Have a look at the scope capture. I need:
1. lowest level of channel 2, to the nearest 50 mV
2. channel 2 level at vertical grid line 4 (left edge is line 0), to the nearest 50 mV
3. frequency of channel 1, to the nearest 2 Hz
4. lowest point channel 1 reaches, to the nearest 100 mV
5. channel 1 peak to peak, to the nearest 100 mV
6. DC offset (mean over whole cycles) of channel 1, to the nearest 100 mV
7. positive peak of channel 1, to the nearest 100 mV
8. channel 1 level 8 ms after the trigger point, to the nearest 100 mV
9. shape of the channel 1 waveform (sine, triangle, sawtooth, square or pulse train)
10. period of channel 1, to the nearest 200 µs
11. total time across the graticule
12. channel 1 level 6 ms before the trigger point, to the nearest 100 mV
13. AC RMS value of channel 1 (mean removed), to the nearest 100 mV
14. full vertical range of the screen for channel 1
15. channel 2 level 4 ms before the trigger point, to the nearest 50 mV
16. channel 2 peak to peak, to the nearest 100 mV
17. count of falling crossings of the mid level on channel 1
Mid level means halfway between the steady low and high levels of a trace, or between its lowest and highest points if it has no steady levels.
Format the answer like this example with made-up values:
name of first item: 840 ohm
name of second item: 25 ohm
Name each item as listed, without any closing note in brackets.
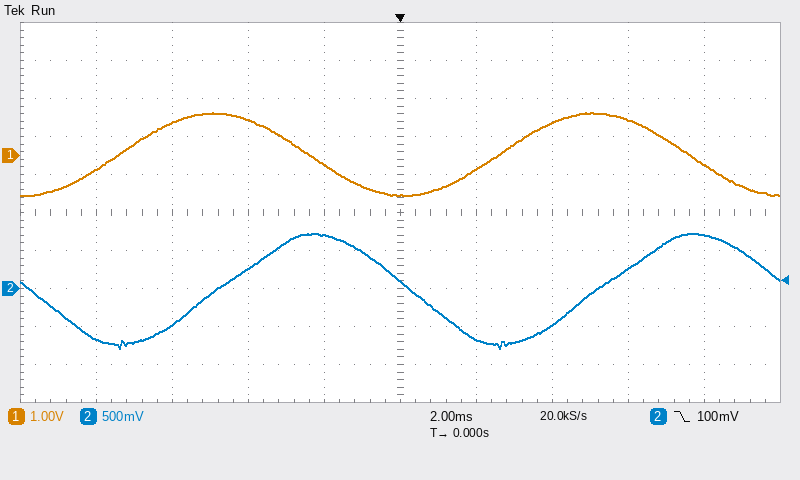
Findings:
lowest level of channel 2, to the nearest 50 mV: -800 mV
channel 2 level at vertical grid line 4 (left edge is line 0), to the nearest 50 mV: 700 mV
frequency of channel 1, to the nearest 2 Hz: 100 Hz
lowest point channel 1 reaches, to the nearest 100 mV: -1.1 V
channel 1 peak to peak, to the nearest 100 mV: 2.2 V
DC offset (mean over whole cycles) of channel 1, to the nearest 100 mV: 0.0 V
positive peak of channel 1, to the nearest 100 mV: 1.1 V
channel 1 level 8 ms after the trigger point, to the nearest 100 mV: -200 mV
shape of the channel 1 waveform: sine
period of channel 1, to the nearest 200 µs: 10.0 ms
total time across the graticule: 20 ms
channel 1 level 6 ms before the trigger point, to the nearest 100 mV: 900 mV
AC RMS value of channel 1 (mean removed), to the nearest 100 mV: 800 mV
full vertical range of the screen for channel 1: 10 V
channel 2 level 4 ms before the trigger point, to the nearest 50 mV: 250 mV
channel 2 peak to peak, to the nearest 100 mV: 1.50 V
count of falling crossings of the mid level on channel 1: 2
